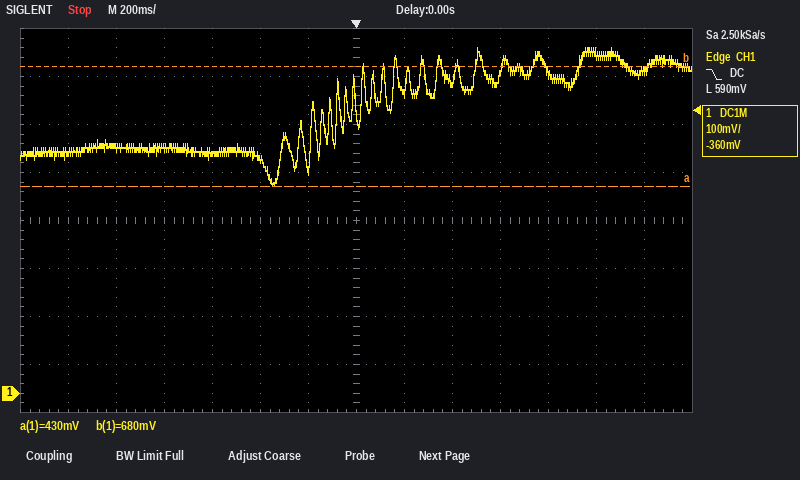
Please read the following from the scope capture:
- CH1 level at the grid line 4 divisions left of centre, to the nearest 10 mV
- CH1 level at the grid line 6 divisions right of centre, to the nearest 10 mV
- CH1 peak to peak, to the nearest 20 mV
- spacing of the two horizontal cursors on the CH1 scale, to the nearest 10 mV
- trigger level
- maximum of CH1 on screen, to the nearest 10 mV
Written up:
510 mV
670 mV
280 mV
250 mV
590 mV
720 mV
